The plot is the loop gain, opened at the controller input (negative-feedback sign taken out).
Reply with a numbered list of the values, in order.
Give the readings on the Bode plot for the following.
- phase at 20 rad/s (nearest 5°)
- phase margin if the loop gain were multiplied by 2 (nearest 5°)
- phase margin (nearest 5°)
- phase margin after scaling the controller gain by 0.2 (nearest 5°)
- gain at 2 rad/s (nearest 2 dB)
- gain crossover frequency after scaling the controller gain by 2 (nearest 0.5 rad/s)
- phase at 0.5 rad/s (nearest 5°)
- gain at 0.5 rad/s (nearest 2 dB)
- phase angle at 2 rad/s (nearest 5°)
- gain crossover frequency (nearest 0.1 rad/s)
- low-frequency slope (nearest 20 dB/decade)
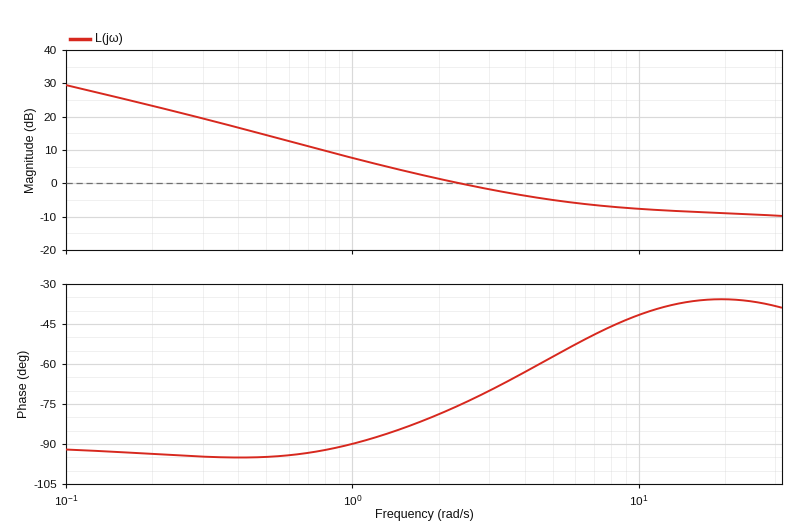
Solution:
1. -35°
2. 130°
3. 105°
4. 85°
5. 2 dB
6. 6.0 rad/s
7. -95°
8. 14 dB
9. -80°
10. 2.4 rad/s
11. -20 dB/decade
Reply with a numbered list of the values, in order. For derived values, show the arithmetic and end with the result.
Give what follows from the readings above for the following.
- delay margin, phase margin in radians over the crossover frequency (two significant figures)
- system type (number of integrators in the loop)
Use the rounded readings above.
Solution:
1. 105 × π / 180 / 2.4 = 0.76 s
2. 1
